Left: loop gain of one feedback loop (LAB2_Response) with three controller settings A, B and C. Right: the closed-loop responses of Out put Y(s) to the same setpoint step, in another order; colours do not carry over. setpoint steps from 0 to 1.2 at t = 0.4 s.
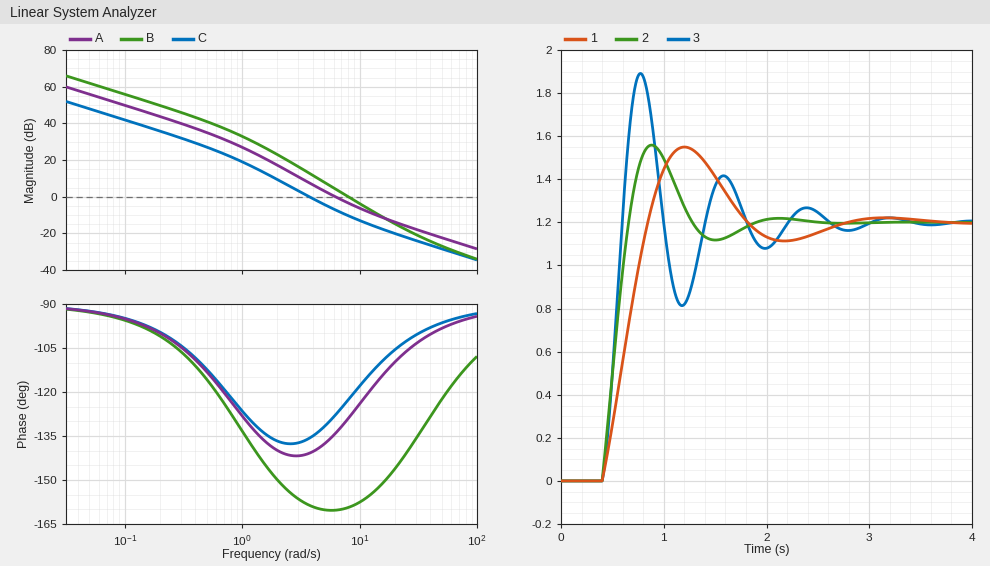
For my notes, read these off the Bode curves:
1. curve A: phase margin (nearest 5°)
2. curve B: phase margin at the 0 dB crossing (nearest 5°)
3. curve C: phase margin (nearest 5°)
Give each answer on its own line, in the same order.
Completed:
45°
20°
45°
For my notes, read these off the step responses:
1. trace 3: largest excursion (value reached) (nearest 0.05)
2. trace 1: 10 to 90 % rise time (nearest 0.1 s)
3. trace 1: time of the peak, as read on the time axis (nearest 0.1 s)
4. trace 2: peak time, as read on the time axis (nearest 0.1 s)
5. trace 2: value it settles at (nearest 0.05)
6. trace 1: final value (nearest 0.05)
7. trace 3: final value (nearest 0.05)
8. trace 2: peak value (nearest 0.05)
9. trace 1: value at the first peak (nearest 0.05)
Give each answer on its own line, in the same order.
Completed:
1.90
0.3 s
1.2 s
0.9 s
1.20
1.20
1.20
1.55
1.55
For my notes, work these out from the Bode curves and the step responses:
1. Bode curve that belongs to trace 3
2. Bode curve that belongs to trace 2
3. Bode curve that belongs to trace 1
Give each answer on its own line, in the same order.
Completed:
B
A
C
